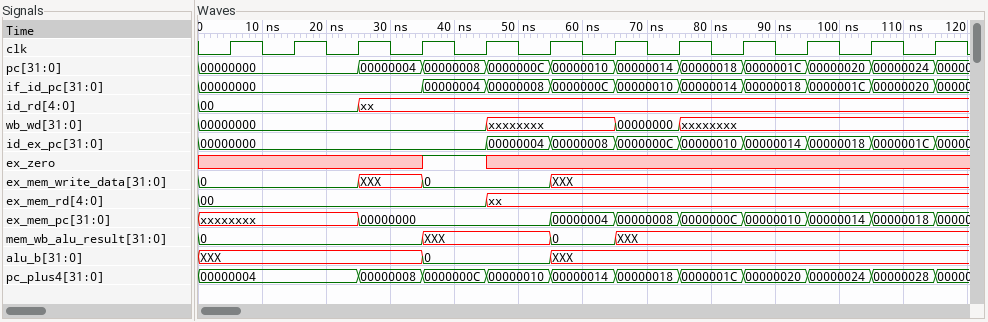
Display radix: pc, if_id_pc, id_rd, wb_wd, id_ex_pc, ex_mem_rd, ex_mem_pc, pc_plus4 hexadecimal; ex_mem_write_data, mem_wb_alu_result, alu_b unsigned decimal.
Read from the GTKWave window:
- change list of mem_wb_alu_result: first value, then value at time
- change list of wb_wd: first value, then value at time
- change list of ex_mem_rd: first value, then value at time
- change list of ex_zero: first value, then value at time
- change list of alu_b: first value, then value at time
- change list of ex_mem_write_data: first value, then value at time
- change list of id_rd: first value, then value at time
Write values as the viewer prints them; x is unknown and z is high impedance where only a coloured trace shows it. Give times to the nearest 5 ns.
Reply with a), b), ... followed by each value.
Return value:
a) 0, XXX at 35 ns, 0 at 55 ns, XXX at 65 ns
b) 00000000, xxxxxxxx at 45 ns, 00000000 at 65 ns, xxxxxxxx at 75 ns
c) 00, xx at 45 ns
d) x, 1 at 35 ns, x at 45 ns
e) XXX, 0 at 35 ns, XXX at 55 ns
f) 0, XXX at 25 ns, 0 at 35 ns, XXX at 55 ns
g) 00, xx at 25 ns
